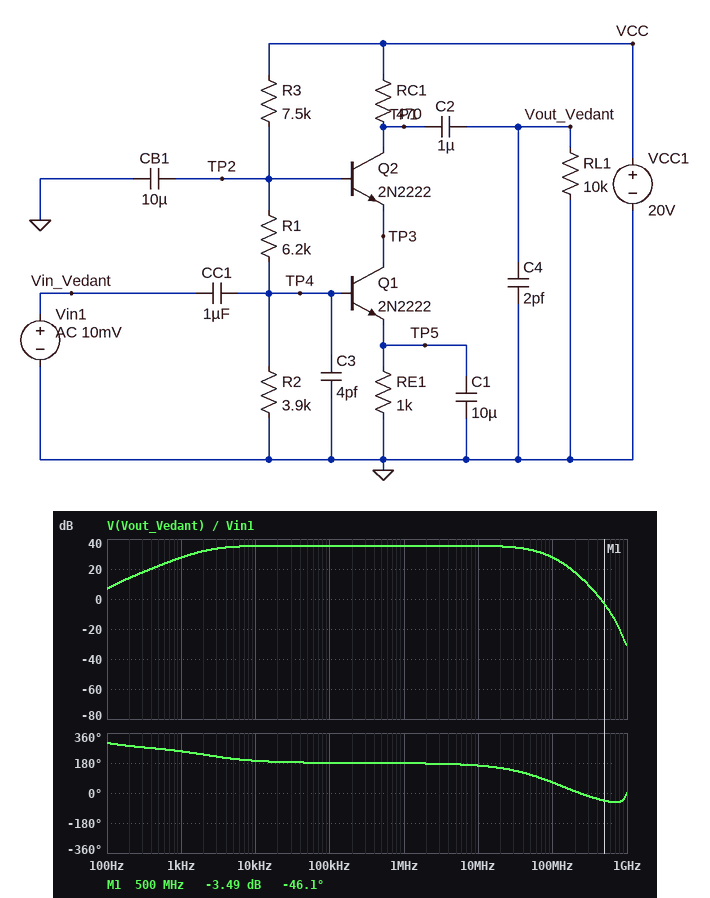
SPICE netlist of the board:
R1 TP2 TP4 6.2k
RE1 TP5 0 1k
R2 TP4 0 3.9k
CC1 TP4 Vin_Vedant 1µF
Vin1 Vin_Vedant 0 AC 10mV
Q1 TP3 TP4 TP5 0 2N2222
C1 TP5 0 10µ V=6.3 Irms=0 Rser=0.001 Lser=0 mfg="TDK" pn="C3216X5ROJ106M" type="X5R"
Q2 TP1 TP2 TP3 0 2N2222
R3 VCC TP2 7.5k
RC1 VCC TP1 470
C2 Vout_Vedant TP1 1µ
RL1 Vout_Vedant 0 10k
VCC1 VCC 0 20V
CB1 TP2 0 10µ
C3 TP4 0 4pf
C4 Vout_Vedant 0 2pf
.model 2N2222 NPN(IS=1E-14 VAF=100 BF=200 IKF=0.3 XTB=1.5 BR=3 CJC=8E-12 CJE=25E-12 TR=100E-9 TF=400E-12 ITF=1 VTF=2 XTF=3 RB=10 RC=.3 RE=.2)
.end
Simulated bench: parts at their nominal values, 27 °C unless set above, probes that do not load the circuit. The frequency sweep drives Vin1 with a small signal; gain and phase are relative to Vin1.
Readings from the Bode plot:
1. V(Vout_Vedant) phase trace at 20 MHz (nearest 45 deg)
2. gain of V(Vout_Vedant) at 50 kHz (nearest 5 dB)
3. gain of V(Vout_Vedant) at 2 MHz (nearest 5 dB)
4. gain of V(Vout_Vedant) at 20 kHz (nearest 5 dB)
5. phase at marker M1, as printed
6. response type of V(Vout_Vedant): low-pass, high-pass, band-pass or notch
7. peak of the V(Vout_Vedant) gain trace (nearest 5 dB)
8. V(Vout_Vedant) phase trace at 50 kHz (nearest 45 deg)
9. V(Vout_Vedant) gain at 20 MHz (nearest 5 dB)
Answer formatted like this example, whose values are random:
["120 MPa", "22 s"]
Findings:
["135 deg", "35 dB", "35 dB", "35 dB", "-46.1 deg", "band-pass", "35 dB", "180 deg", "35 dB"]
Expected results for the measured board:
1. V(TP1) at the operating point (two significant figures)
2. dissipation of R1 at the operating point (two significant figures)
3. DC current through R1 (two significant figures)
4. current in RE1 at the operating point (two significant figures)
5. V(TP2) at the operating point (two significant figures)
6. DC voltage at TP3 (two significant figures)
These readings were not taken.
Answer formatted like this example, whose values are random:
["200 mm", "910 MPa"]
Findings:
["18 V", "8.0 mW", "1.1 mA", "3.7 mA", "11 V", "11 V"]
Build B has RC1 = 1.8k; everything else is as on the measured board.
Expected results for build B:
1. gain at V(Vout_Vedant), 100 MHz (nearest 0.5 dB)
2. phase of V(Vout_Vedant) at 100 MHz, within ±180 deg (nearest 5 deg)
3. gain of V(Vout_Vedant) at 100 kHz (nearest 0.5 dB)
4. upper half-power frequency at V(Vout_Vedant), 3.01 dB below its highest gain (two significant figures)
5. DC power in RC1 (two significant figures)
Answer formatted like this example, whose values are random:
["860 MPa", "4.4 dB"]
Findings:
["27.0 dB", "40 deg", "46.0 dB", "14 MHz", "24 mW"]
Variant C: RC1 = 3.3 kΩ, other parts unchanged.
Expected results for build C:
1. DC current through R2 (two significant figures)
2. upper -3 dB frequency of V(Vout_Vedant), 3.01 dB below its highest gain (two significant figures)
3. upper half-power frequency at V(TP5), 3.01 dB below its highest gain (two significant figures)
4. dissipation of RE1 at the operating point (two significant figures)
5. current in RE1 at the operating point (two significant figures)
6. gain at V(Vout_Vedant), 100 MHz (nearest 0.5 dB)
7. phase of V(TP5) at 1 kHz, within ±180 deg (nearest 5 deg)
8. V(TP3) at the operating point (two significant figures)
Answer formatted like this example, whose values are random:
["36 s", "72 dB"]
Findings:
["1.0 mA", "570 kHz", "2.2 kHz", "11 mW", "3.3 mA", "0 dB", "-20 deg", "9.8 V"]
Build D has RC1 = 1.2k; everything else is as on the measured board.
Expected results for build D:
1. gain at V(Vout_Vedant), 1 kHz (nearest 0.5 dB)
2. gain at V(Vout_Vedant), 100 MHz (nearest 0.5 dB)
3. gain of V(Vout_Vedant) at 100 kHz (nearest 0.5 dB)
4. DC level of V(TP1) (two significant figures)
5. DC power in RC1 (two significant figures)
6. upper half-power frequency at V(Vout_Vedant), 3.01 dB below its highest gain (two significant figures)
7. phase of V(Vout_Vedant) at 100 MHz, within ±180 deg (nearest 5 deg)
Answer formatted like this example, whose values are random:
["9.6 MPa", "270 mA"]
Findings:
["35.0 dB", "28.0 dB", "43.0 dB", "16 V", "16 mW", "23 MHz", "45 deg"]
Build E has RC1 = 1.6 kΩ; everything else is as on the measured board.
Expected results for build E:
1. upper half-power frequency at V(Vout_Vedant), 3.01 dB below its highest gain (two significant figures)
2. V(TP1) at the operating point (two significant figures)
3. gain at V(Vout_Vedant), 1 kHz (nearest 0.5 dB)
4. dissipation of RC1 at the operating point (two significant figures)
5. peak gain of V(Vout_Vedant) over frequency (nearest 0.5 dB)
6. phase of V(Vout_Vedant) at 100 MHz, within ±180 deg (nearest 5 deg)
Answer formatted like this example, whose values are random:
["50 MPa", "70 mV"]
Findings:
["17 MHz", "14 V", "37.5 dB", "21 mW", "45.5 dB", "40 deg"]
